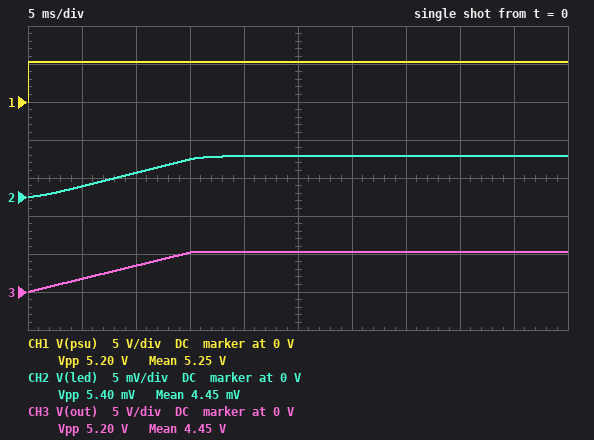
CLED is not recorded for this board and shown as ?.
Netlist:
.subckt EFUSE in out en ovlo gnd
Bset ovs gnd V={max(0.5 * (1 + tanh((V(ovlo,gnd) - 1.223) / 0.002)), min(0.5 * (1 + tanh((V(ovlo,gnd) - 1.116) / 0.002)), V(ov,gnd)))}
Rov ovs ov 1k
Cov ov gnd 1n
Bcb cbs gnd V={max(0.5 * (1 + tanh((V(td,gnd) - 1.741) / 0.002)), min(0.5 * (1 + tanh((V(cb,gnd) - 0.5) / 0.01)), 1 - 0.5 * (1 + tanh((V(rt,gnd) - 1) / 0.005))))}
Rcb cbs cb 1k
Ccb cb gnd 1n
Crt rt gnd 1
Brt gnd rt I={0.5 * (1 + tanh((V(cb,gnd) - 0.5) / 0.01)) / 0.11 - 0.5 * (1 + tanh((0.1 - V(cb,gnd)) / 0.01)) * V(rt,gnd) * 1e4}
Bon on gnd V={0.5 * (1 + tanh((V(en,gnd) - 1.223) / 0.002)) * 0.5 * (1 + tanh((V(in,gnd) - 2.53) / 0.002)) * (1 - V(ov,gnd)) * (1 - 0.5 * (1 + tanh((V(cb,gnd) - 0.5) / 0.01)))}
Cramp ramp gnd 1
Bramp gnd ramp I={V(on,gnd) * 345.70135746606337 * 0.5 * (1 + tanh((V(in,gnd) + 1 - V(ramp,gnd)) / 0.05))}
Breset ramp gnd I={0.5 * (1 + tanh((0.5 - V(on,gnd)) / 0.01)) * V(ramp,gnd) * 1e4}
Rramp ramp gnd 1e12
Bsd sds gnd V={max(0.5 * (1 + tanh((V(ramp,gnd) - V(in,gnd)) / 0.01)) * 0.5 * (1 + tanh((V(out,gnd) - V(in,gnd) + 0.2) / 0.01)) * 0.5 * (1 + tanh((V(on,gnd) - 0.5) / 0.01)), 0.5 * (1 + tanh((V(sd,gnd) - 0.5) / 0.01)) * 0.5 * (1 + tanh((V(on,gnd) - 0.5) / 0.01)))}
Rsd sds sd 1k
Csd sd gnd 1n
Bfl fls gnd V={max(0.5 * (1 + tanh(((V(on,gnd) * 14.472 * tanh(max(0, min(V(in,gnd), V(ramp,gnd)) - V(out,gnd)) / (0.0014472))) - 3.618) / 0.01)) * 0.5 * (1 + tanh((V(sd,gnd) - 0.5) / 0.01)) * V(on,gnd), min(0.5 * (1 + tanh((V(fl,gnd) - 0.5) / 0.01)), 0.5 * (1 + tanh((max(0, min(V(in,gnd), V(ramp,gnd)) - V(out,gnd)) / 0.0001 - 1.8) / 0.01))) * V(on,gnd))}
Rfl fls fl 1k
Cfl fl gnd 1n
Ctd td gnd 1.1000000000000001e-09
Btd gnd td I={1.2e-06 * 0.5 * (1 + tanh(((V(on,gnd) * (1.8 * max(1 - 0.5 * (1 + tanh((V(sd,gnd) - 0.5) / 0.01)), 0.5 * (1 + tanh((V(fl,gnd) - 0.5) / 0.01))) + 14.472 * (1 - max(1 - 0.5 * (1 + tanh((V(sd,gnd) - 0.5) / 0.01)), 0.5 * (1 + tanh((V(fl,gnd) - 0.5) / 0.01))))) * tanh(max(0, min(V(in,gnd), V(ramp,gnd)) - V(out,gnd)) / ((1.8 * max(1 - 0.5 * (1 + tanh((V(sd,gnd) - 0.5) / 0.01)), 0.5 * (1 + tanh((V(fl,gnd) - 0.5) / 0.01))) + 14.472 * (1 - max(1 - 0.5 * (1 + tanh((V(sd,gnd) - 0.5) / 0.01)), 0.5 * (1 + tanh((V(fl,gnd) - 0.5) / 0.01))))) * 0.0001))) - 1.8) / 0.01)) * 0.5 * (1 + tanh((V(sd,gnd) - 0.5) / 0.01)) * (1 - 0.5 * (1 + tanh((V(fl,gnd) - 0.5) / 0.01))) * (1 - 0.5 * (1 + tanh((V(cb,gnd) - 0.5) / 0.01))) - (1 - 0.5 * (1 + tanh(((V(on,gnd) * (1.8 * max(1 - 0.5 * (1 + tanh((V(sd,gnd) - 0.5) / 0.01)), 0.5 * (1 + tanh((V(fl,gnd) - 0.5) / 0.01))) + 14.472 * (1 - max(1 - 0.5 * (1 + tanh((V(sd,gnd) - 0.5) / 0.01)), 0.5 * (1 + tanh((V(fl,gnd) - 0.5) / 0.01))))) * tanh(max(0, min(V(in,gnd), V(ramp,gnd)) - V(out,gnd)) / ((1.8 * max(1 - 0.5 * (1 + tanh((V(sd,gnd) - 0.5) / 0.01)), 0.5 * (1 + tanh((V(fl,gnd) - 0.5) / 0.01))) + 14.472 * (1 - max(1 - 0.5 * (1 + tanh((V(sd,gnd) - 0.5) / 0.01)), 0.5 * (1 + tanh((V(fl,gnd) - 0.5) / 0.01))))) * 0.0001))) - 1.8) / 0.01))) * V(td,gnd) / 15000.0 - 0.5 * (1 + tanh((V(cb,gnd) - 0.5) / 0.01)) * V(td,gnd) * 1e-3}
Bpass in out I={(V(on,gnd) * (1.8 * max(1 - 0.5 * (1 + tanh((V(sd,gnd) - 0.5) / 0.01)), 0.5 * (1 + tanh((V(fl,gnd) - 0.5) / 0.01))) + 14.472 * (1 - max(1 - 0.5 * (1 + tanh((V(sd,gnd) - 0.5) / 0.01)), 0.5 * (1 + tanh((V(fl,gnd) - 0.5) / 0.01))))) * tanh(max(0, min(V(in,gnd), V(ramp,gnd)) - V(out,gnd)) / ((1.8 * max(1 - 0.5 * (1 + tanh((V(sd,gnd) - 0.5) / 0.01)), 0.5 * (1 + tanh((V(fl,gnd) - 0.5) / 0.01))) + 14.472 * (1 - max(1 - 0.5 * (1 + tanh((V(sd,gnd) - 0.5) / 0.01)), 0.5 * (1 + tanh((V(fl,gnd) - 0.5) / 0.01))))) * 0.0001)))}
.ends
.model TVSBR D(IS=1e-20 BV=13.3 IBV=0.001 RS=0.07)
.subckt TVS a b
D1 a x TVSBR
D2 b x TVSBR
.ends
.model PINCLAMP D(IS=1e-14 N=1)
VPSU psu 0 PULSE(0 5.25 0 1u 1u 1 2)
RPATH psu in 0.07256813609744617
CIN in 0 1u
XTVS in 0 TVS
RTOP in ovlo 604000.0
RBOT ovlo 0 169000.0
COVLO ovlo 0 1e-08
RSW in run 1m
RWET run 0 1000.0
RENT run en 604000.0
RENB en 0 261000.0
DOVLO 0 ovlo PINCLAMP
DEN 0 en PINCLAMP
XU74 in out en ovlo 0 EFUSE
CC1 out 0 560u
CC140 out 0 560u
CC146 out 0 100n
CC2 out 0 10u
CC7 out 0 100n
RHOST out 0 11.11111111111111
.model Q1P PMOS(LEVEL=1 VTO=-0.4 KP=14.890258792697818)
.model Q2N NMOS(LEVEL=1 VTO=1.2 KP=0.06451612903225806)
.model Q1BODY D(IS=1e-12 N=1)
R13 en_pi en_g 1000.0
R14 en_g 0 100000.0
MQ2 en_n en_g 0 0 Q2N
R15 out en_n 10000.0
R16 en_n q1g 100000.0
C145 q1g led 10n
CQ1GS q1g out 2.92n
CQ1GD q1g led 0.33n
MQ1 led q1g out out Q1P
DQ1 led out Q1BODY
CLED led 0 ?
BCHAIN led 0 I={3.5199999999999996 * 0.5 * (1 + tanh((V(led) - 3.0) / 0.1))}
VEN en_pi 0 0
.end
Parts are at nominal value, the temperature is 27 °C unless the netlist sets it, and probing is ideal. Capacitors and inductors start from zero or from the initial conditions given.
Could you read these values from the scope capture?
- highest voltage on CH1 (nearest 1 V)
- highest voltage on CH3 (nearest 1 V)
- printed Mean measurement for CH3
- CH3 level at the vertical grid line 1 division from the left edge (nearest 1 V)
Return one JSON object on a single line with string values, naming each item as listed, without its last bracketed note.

{"highest voltage on CH1": "5 V", "highest voltage on CH3": "5 V", "printed Mean measurement for CH3": "4.45 V", "CH3 level at the vertical grid line 1 division from the left edge": "2 V"}
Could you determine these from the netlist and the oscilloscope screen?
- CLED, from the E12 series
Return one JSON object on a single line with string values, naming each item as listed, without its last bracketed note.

{"CLED, from the E12 series": "10 µF"}
